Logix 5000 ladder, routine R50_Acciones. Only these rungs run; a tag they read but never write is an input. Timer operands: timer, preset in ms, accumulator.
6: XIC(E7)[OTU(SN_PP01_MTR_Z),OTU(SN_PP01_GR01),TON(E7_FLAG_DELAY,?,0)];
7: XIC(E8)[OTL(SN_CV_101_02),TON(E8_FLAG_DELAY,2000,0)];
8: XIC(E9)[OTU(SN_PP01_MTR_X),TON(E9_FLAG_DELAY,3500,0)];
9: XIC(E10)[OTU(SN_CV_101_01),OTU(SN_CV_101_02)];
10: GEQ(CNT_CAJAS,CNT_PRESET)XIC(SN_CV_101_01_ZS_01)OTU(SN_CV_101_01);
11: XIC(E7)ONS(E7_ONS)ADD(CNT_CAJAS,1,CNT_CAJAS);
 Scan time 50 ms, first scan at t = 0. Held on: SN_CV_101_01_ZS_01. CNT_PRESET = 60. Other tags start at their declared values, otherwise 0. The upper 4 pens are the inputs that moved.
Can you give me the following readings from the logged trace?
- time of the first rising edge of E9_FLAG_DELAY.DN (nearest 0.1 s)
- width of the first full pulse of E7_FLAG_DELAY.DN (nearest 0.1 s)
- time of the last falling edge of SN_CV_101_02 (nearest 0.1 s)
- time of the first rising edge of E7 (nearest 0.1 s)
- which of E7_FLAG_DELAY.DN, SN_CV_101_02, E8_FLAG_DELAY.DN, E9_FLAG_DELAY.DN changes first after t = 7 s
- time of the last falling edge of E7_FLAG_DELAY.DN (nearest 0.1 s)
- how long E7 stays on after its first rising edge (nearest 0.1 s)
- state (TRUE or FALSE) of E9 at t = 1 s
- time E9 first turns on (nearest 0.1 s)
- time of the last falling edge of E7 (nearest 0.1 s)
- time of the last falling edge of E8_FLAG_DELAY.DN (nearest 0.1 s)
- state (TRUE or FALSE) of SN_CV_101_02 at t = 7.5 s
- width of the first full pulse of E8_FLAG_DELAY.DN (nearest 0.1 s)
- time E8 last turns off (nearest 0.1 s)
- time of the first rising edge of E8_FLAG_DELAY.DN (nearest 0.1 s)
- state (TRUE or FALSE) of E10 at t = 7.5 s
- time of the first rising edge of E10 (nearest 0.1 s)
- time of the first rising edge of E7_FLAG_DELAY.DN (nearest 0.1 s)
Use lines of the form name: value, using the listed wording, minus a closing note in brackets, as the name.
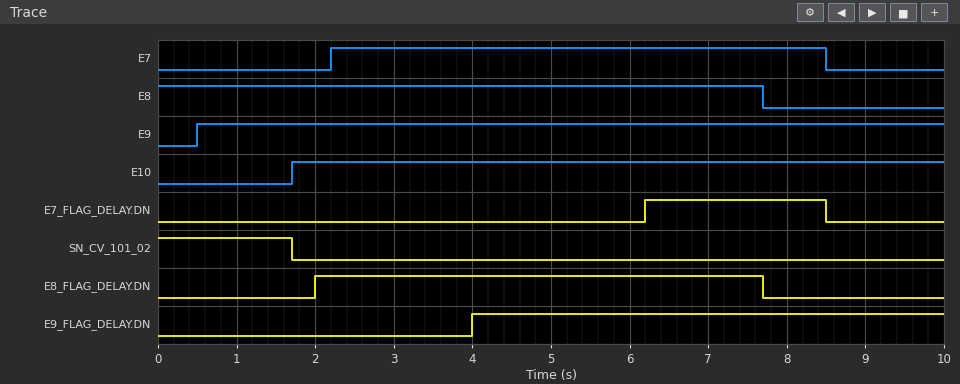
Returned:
time of the first rising edge of E9_FLAG_DELAY.DN: 4.0 s
width of the first full pulse of E7_FLAG_DELAY.DN: 2.3 s
time of the last falling edge of SN_CV_101_02: 1.7 s
time of the first rising edge of E7: 2.2 s
which of E7_FLAG_DELAY.DN, SN_CV_101_02, E8_FLAG_DELAY.DN, E9_FLAG_DELAY.DN changes first after t = 7 s: E8_FLAG_DELAY.DN
time of the last falling edge of E7_FLAG_DELAY.DN: 8.5 s
how long E7 stays on after its first rising edge: 6.3 s
state (TRUE or FALSE) of E9 at t = 1 s: TRUE
time E9 first turns on: 0.5 s
time of the last falling edge of E7: 8.5 s
time of the last falling edge of E8_FLAG_DELAY.DN: 7.7 s
state (TRUE or FALSE) of SN_CV_101_02 at t = 7.5 s: FALSE
width of the first full pulse of E8_FLAG_DELAY.DN: 5.7 s
time E8 last turns off: 7.7 s
time of the first rising edge of E8_FLAG_DELAY.DN: 2.0 s
state (TRUE or FALSE) of E10 at t = 7.5 s: TRUE
time of the first rising edge of E10: 1.7 s
time of the first rising edge of E7_FLAG_DELAY.DN: 6.2 s
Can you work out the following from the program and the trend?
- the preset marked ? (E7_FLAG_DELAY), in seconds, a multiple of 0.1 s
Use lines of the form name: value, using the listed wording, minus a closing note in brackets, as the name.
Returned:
the preset marked ? (E7_FLAG_DELAY), in seconds, a multiple of 0.1 s: 4.0 s
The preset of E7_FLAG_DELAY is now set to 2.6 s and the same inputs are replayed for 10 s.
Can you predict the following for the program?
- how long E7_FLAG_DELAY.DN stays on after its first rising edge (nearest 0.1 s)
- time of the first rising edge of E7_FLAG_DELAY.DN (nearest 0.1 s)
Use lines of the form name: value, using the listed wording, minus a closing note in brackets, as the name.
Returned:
how long E7_FLAG_DELAY.DN stays on after its first rising edge: 3.7 s
time of the first rising edge of E7_FLAG_DELAY.DN: 4.8 s
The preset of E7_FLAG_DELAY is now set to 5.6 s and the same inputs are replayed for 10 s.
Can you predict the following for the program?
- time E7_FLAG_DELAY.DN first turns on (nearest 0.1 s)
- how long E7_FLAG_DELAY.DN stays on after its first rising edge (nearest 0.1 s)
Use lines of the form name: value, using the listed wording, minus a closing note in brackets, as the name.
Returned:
time E7_FLAG_DELAY.DN first turns on: 7.8 s
how long E7_FLAG_DELAY.DN stays on after its first rising edge: 0.7 s
